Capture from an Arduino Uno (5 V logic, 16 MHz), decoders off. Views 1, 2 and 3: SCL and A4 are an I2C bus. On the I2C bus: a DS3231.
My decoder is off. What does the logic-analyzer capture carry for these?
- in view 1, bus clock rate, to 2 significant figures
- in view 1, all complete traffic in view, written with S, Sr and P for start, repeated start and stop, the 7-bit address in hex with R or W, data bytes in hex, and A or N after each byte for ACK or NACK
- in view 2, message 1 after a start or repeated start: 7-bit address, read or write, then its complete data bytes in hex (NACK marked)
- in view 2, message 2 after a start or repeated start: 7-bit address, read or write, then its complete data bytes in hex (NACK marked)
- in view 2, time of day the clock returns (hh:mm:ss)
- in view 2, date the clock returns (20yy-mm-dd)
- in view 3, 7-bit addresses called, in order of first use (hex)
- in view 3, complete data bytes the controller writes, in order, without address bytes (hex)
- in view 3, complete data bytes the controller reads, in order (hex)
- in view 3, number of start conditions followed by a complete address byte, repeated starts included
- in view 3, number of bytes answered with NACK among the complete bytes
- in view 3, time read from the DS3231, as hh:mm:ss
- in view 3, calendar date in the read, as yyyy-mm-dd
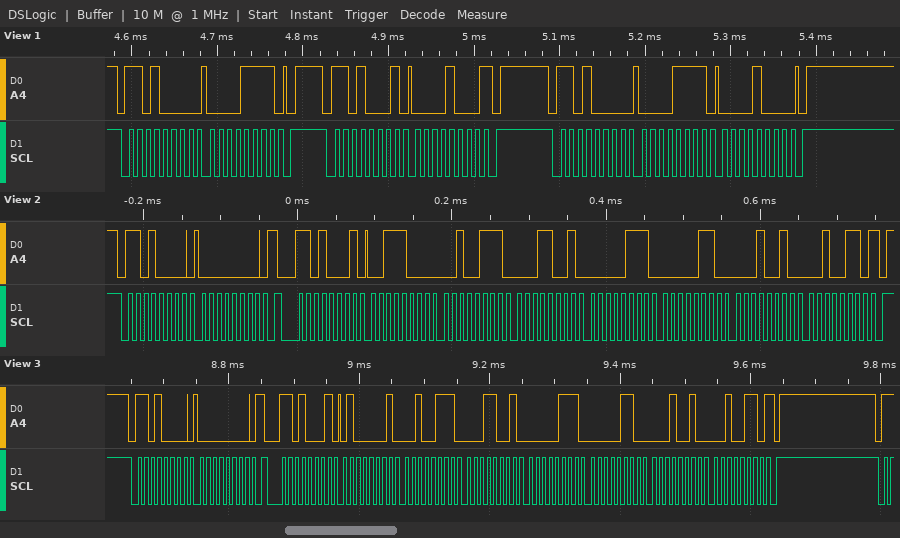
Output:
100 kHz
S 68W A 0F A P S 68R A 08 N P S 68W A 0F A 08 A P
0x68 write: 00
0x68 read: 38 27 19 07 06 12 26 NACK
19:27:38
2026-12-06
0x68
00
41 27 19 07 06 12 26
2
1
19:27:41
2026-12-06
